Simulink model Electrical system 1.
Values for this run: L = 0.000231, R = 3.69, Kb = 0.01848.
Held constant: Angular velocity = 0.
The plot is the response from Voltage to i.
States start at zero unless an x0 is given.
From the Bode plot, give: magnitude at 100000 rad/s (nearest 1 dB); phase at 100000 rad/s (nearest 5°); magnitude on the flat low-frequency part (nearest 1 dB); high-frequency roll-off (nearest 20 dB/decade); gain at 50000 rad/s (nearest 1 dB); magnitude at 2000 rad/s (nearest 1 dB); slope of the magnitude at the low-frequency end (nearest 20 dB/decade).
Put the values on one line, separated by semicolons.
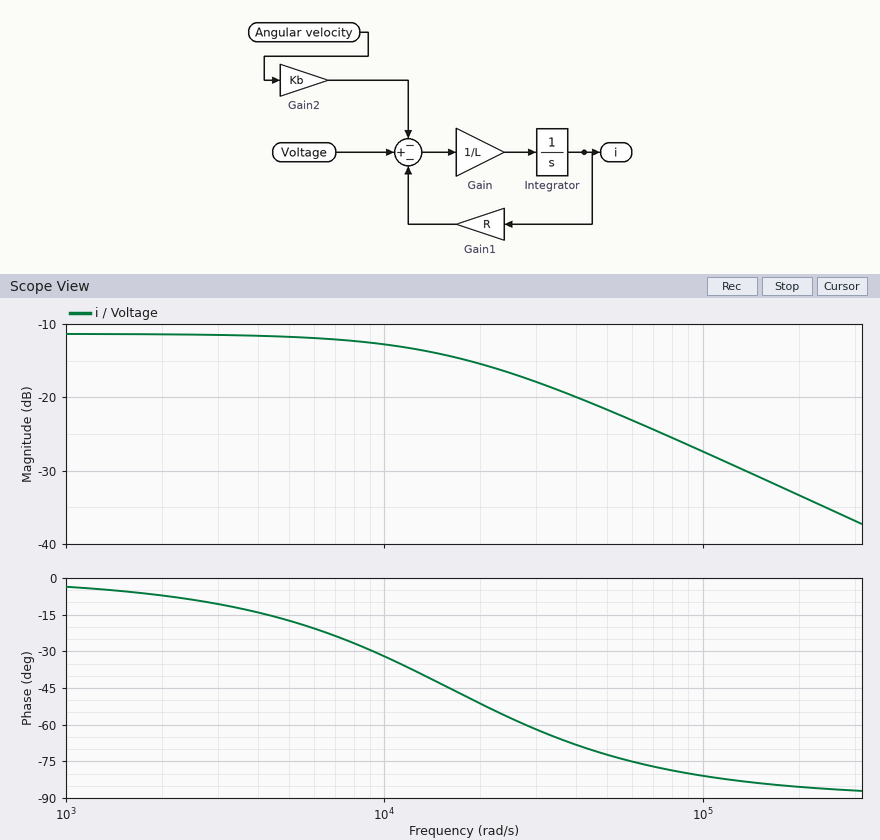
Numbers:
-27 dB; -80°; -11 dB; -20 dB/decade; -22 dB; -11 dB; 0 dB/decade
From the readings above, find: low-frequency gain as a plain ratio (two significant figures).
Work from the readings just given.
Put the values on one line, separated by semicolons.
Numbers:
0.28
